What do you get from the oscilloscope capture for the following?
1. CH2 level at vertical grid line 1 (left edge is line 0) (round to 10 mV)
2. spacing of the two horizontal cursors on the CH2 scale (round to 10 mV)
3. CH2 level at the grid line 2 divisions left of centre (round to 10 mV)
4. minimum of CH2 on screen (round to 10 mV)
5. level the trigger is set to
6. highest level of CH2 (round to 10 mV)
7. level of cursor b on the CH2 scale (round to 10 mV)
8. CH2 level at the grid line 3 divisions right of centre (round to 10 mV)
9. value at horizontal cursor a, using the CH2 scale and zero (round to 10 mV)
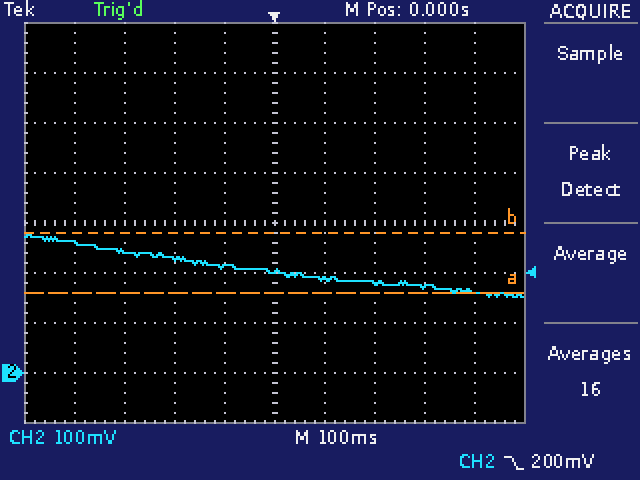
260 mV
120 mV
230 mV
150 mV
200 mV
280 mV
280 mV
170 mV
160 mV
